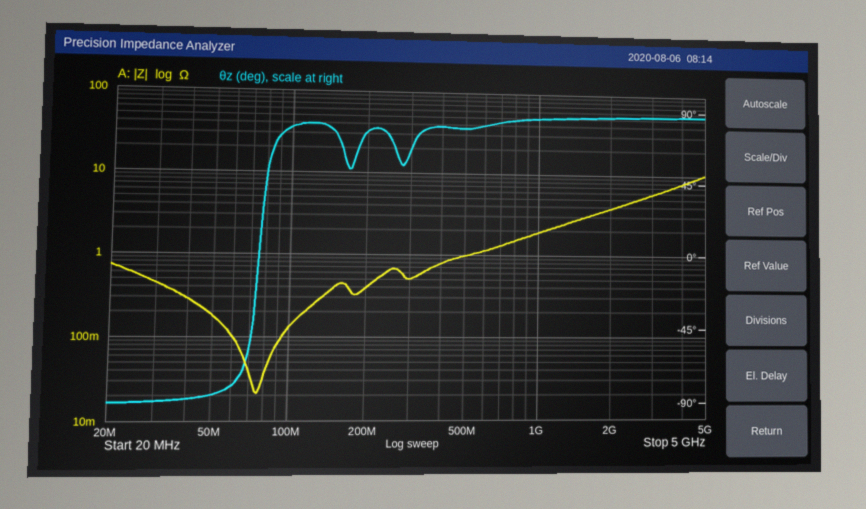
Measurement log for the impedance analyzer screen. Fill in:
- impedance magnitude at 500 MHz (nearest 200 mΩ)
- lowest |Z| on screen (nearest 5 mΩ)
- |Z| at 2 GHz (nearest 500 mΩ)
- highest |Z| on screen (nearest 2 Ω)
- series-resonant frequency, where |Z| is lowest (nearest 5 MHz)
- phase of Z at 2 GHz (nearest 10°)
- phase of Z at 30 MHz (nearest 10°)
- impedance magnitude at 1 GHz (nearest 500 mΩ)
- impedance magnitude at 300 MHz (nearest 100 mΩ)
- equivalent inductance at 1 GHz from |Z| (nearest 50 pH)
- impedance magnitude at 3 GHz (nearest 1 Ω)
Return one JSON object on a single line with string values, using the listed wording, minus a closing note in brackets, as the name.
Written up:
{"impedance magnitude at 500 MHz": "1.0 Ω", "lowest |Z| on screen": "20 mΩ", "|Z| at 2 GHz": "4.0 Ω", "highest |Z| on screen": "10 Ω", "series-resonant frequency, where |Z| is lowest": "75 MHz", "phase of Z at 2 GHz": "90°", "phase of Z at 30 MHz": "-90°", "impedance magnitude at 1 GHz": "2.0 Ω", "impedance magnitude at 300 MHz": "500 mΩ", "equivalent inductance at 1 GHz from |Z|": "300 pH", "impedance magnitude at 3 GHz": "6 Ω"}
